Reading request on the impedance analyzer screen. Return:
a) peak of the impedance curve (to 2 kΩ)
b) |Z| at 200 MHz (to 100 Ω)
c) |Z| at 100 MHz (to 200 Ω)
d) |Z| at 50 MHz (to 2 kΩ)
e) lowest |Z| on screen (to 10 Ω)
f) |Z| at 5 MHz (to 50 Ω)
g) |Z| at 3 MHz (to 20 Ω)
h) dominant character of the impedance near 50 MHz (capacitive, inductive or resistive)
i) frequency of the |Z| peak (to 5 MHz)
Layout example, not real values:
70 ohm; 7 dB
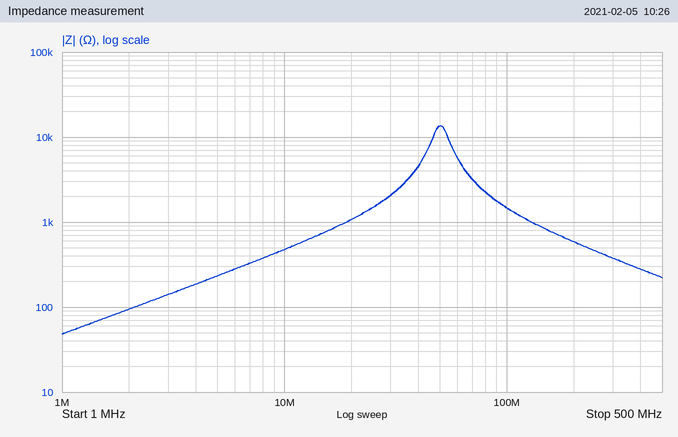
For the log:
14 kΩ; 600 Ω; 1.4 kΩ; 14 kΩ; 50 Ω; 250 Ω; 140 Ω; resistive; 50 MHz
